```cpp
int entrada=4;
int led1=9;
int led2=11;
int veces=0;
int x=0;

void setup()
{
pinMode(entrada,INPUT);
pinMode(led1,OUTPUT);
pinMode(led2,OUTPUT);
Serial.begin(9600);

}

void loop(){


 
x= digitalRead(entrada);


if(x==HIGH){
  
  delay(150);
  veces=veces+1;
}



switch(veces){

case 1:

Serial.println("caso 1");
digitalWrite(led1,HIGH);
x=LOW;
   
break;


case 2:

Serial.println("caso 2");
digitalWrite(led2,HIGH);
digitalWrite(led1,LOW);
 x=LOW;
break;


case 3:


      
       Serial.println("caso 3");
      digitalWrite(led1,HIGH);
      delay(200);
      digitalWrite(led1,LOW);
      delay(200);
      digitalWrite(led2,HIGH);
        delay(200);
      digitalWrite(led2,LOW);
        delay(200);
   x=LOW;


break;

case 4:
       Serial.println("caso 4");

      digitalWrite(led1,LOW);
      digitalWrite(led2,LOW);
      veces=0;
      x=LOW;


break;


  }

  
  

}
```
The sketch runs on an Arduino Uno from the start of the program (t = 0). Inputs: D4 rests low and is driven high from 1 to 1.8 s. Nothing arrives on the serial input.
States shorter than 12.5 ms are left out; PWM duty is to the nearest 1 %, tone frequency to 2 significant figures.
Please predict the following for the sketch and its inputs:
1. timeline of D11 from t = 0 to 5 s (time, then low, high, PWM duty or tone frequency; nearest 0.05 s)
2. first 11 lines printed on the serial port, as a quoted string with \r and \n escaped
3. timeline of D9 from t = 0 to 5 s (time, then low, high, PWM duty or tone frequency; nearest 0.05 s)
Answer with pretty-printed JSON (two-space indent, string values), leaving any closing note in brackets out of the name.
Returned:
{
  "timeline of D11 from t = 0 to 5 s": "0 s low; 1.3 s high; 2.05 s low; 2.65 s high; 2.85 s low; 3.45 s high; 3.65 s low; 4.25 s high; 4.45 s low",
  "first 11 lines printed on the serial port, as a quoted string with \\r and \\n escaped": "\"caso 1\\r\\ncaso 2\\r\\ncaso 3\\r\\ncaso 3\\r\\ncaso 3\\r\\ncaso 3\\r\\ncaso 3\\r\\ncaso 3\\r\\ncaso 3\\r\\ncaso 3\\r\\ncaso 3\\r\\n\"",
  "timeline of D9 from t = 0 to 5 s": "0 s low; 1.15 s high; 1.3 s low; 1.45 s high; 1.65 s low; 2.25 s high; 2.45 s low; 3.05 s high; 3.25 s low; 3.85 s high; 4.05 s low; 4.65 s high; 4.85 s low"
}
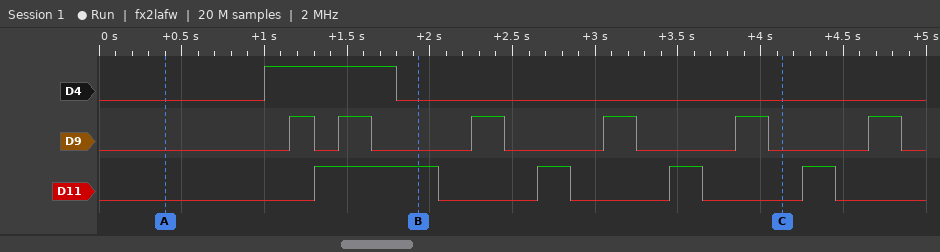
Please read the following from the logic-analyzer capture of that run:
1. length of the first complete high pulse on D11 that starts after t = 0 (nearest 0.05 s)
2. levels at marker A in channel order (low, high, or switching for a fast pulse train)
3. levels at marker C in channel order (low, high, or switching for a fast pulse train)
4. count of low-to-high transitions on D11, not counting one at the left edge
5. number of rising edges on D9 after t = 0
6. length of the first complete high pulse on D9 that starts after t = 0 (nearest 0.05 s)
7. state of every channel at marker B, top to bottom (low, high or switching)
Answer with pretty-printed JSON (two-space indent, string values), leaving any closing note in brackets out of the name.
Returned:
{
  "length of the first complete high pulse on D11 that starts after t = 0": "0.75 s",
  "levels at marker A in channel order": "D4 low, D9 low, D11 low",
  "levels at marker C in channel order": "D4 low, D9 low, D11 low",
  "count of low-to-high transitions on D11, not counting one at the left edge": "4",
  "number of rising edges on D9 after t = 0": "6",
  "length of the first complete high pulse on D9 that starts after t = 0": "0.15 s",
  "state of every channel at marker B, top to bottom": "D4 low, D9 low, D11 high"
}
